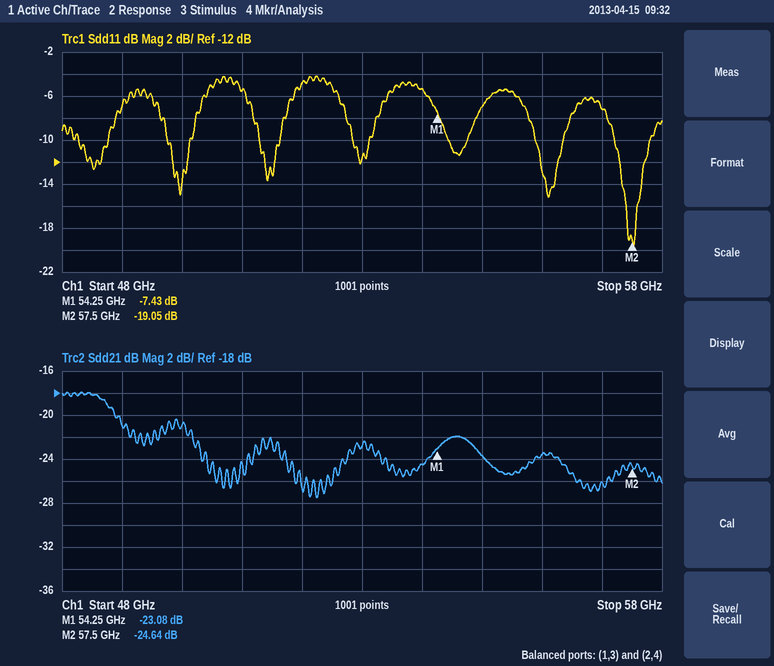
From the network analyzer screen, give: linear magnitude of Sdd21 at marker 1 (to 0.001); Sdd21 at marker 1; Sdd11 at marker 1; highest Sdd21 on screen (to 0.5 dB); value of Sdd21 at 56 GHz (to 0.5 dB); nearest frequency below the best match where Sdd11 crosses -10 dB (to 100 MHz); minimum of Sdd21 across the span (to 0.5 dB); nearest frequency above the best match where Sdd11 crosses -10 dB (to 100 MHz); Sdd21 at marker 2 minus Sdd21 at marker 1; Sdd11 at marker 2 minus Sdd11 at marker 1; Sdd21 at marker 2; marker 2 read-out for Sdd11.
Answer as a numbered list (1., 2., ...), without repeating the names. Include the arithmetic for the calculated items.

1. 10^(-23.08/20) ≈ 0.070
2. -23.08 dB
3. -7.43 dB
4. -18.0 dB
5. -23.5 dB
6. 57.2 GHz
7. -27.5 dB
8. 57.8 GHz
9. -24.64 − (-23.08) = -1.56 dB
10. -19.05 − (-7.43) = -11.62 dB
11. -24.64 dB
12. -19.05 dB
